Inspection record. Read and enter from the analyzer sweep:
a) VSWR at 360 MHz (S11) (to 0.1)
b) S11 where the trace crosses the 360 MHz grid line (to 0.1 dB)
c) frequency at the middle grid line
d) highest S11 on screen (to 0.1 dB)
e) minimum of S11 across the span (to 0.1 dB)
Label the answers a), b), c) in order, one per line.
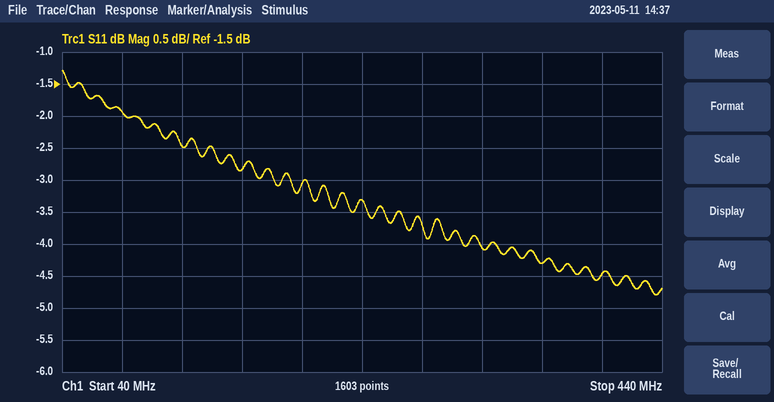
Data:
a) 4.1
b) -4.3 dB
c) 240 MHz
d) -1.3 dB
e) -4.8 dB
